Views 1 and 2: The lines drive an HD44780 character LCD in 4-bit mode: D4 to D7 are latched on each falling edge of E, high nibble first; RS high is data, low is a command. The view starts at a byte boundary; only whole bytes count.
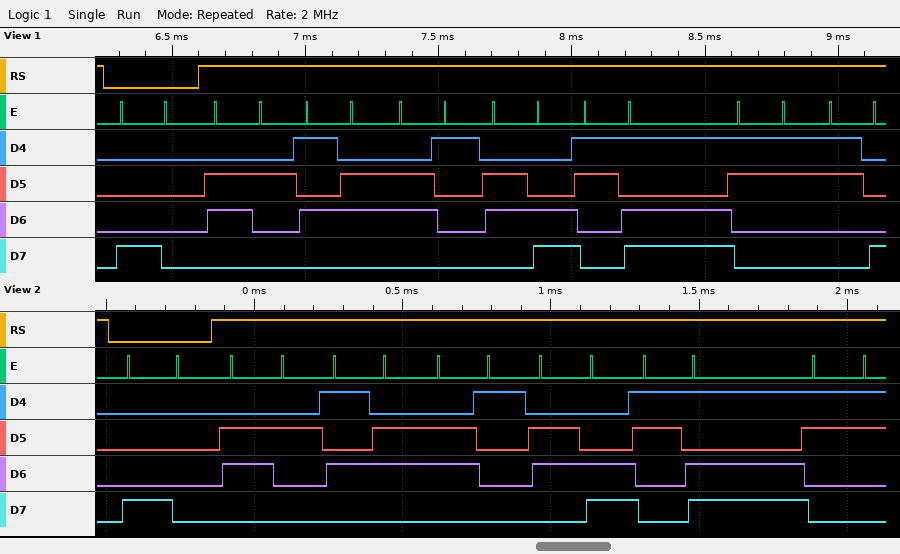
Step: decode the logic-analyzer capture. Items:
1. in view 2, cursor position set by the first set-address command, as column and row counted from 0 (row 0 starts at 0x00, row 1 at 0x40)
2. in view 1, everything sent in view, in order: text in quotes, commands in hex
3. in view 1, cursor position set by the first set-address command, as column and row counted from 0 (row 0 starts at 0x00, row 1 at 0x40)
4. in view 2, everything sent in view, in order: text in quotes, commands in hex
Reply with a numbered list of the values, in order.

1. column 0, row 0
2. 0x80 "bVal=38"
3. column 0, row 0
4. 0x80 "bVal=3"
